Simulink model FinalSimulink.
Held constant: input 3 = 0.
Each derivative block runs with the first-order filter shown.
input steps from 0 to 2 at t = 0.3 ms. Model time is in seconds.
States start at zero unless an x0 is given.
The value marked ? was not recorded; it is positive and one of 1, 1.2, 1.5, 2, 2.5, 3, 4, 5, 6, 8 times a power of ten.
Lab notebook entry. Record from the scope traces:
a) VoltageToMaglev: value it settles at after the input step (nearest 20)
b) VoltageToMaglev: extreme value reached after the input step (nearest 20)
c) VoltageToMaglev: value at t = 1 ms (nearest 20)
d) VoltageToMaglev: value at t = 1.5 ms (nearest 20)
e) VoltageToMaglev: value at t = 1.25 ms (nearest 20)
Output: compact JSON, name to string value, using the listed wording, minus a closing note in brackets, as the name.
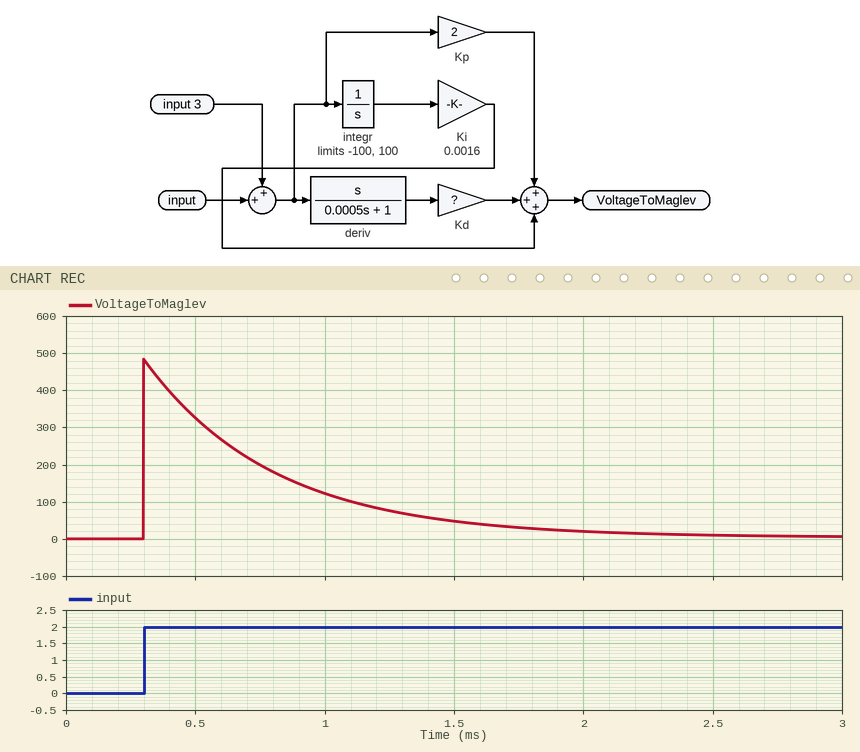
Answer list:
{"VoltageToMaglev: value it settles at after the input step": "0", "VoltageToMaglev: extreme value reached after the input step": "480", "VoltageToMaglev: value at t = 1 ms": "120", "VoltageToMaglev: value at t = 1.5 ms": "40", "VoltageToMaglev: value at t = 1.25 ms": "80"}
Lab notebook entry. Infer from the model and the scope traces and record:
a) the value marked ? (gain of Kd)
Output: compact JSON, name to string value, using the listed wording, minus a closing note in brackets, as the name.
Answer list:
{"the value marked ?": "0.12"}
